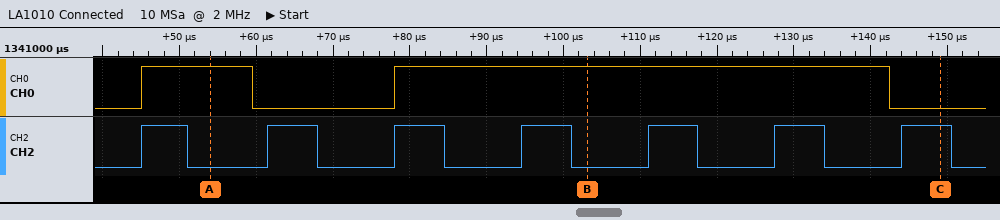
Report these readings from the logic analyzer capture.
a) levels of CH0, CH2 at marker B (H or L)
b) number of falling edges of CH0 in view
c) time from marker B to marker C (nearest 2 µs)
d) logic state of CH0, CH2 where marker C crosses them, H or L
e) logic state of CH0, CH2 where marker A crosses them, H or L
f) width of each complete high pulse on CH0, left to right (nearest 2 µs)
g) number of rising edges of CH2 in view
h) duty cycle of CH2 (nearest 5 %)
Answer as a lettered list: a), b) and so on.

a) CH0=H, CH2=L
b) 2
c) 46 µs
d) CH0=L, CH2=H
e) CH0=H, CH2=L
f) 14 µs, 64 µs
g) 7
h) 40 %
